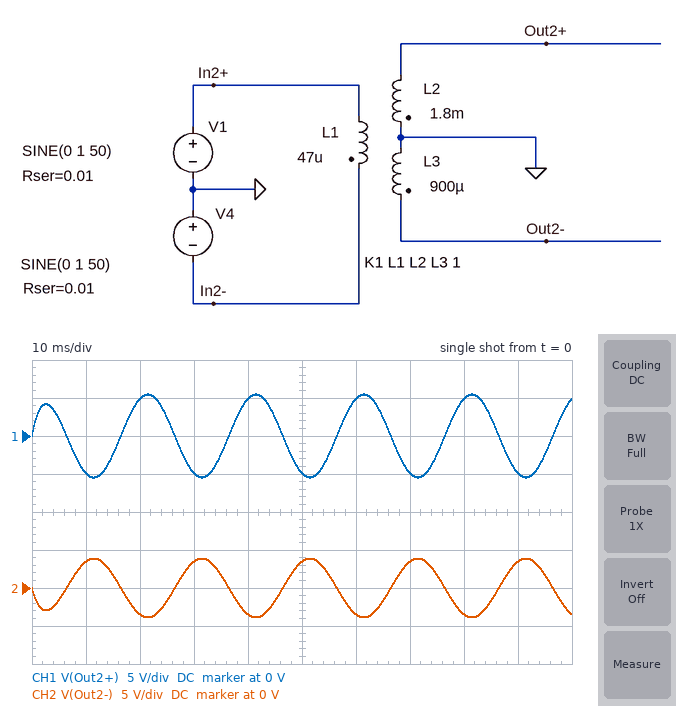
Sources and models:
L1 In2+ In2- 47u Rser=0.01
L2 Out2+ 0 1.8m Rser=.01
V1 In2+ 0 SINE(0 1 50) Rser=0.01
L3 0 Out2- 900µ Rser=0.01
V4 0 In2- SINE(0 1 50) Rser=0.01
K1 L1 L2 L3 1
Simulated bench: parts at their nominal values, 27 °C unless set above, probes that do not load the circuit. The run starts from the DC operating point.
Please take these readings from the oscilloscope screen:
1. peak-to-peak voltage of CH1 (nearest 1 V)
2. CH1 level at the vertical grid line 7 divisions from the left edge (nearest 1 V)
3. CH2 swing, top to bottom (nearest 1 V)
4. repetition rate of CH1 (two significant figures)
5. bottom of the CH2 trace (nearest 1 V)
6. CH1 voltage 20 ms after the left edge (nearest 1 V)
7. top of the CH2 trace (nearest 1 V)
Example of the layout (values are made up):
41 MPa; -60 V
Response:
11 V; -5 V; 8 V; 50 Hz; -4 V; 5 V; 4 V
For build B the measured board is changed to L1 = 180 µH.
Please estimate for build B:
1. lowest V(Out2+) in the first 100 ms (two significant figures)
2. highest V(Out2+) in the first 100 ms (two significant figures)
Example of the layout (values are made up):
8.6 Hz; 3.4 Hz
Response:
-5.9 V; 5.6 V
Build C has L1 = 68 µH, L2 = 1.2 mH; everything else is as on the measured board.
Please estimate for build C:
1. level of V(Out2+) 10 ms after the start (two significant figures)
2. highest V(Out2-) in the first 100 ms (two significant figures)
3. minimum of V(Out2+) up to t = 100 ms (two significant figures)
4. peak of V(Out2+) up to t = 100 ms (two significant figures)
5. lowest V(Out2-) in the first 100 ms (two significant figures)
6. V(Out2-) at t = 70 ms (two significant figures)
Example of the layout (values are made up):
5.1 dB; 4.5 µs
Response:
-4.0 V; 4.2 V; -4.9 V; 4.9 V; -4.2 V; 3.4 V
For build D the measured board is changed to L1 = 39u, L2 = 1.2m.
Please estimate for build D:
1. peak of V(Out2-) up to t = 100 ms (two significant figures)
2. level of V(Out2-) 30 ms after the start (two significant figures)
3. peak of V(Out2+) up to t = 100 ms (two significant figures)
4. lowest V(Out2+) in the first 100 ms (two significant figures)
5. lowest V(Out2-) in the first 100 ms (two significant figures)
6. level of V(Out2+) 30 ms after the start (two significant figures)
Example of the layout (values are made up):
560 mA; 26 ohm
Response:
3.6 V; 3.4 V; 4.2 V; -4.2 V; -3.6 V; -3.9 V
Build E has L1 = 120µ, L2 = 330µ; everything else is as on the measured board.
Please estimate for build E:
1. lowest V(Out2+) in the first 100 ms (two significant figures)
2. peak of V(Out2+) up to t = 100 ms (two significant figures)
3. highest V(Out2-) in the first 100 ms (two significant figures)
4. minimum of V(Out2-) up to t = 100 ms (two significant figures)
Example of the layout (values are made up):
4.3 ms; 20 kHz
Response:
-2.7 V; 2.6 V; 4.4 V; -4.3 V
